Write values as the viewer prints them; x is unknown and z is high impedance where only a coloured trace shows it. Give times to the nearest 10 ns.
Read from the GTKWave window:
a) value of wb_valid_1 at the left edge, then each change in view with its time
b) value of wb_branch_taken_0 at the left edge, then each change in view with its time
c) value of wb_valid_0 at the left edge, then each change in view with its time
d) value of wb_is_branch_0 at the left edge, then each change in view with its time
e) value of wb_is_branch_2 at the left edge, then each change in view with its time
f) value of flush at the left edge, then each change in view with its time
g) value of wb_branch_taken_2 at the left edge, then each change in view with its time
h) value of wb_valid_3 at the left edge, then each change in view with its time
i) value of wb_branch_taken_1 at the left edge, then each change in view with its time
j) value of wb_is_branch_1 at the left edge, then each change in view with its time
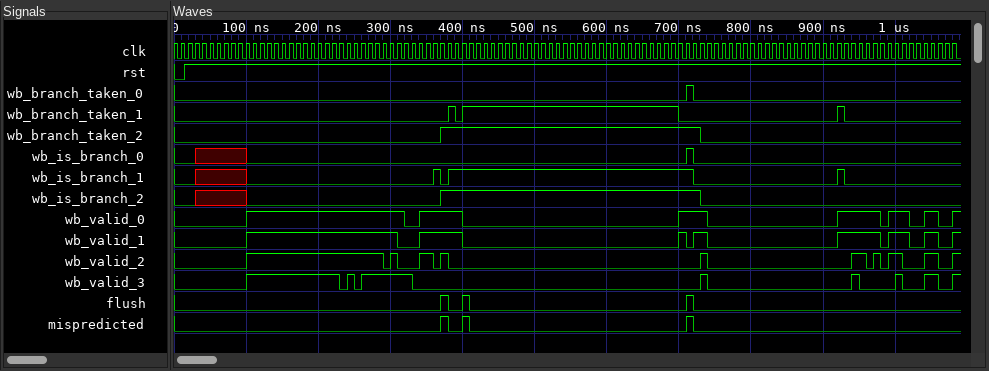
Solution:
0, 1 at 100 ns, 0 at 310 ns, 1 at 340 ns, 0 at 400 ns, 1 at 700 ns, 0 at 710 ns, 1 at 720 ns, 0 at 740 ns, 1 at 920 ns, 0 at 980 ns, 1 at 990 ns, 0 at 1020 ns, 1 at 1040 ns, 0 at 1060 ns, 1 at 1080 ns
0, 1 at 710 ns, 0 at 720 ns
0, 1 at 100 ns, 0 at 320 ns, 1 at 340 ns, 0 at 400 ns, 1 at 700 ns, 0 at 740 ns, 1 at 920 ns, 0 at 980 ns, 1 at 990 ns, 0 at 1020 ns, 1 at 1040 ns, 0 at 1060 ns, 1 at 1080 ns
0, x at 30 ns, 0 at 100 ns, 1 at 710 ns, 0 at 720 ns
0, x at 30 ns, 0 at 100 ns, 1 at 370 ns, 0 at 730 ns
0, 1 at 370 ns, 0 at 380 ns, 1 at 400 ns, 0 at 410 ns, 1 at 710 ns, 0 at 720 ns
0, 1 at 370 ns, 0 at 730 ns
0, 1 at 100 ns, 0 at 230 ns, 1 at 240 ns, 0 at 250 ns, 1 at 260 ns, 0 at 330 ns, 1 at 730 ns, 0 at 740 ns, 1 at 940 ns, 0 at 950 ns, 1 at 1000 ns, 0 at 1010 ns, 1 at 1040 ns, 0 at 1060 ns, 1 at 1080 ns
0, 1 at 380 ns, 0 at 390 ns, 1 at 400 ns, 0 at 700 ns, 1 at 920 ns, 0 at 930 ns
0, x at 30 ns, 0 at 100 ns, 1 at 360 ns, 0 at 370 ns, 1 at 380 ns, 0 at 720 ns, 1 at 920 ns, 0 at 930 ns
